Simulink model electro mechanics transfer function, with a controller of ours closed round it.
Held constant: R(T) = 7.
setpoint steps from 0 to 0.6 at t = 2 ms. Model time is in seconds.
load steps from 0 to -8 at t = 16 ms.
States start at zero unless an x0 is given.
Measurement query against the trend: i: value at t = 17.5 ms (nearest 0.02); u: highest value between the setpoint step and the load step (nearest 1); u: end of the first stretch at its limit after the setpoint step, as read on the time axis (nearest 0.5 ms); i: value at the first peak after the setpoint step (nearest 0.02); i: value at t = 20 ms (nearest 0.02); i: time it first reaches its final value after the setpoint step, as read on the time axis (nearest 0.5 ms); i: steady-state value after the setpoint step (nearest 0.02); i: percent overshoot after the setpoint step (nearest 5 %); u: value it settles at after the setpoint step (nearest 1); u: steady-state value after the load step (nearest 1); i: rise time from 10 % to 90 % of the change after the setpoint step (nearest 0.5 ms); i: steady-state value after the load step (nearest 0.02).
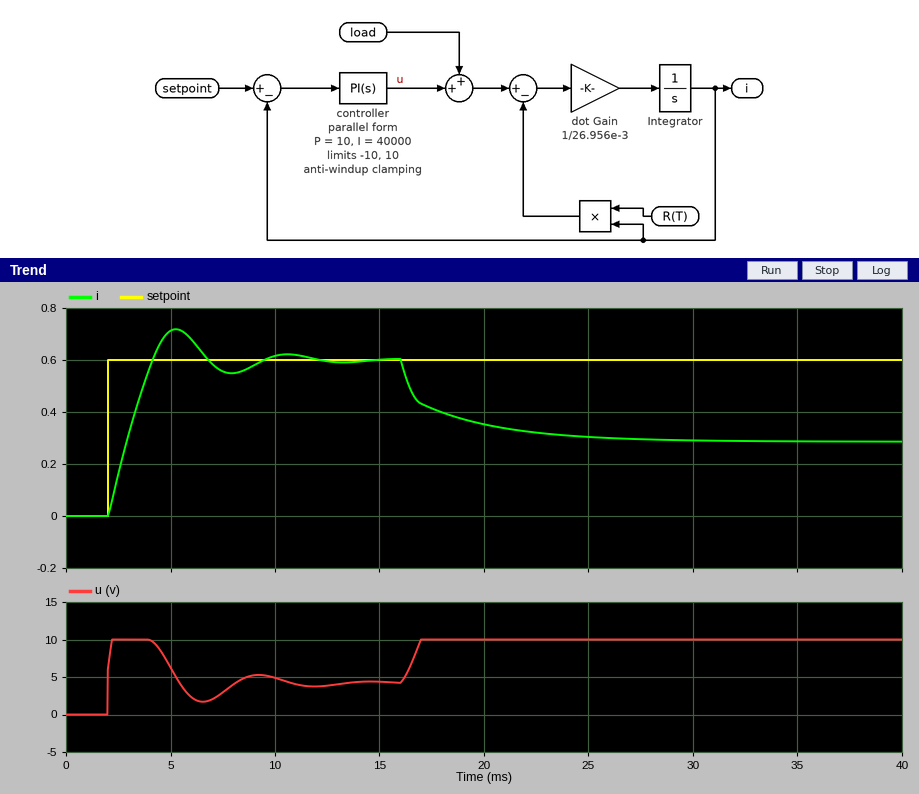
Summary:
0.42
10
4.0 ms
0.72
0.36
4.0 ms
0.60
20 %
4
10
1.5 ms
0.28
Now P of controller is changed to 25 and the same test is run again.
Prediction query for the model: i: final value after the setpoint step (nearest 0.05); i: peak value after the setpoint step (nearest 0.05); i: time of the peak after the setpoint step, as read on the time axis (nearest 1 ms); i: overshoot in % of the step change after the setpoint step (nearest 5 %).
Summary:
0.60
0.65
5 ms
10 %
